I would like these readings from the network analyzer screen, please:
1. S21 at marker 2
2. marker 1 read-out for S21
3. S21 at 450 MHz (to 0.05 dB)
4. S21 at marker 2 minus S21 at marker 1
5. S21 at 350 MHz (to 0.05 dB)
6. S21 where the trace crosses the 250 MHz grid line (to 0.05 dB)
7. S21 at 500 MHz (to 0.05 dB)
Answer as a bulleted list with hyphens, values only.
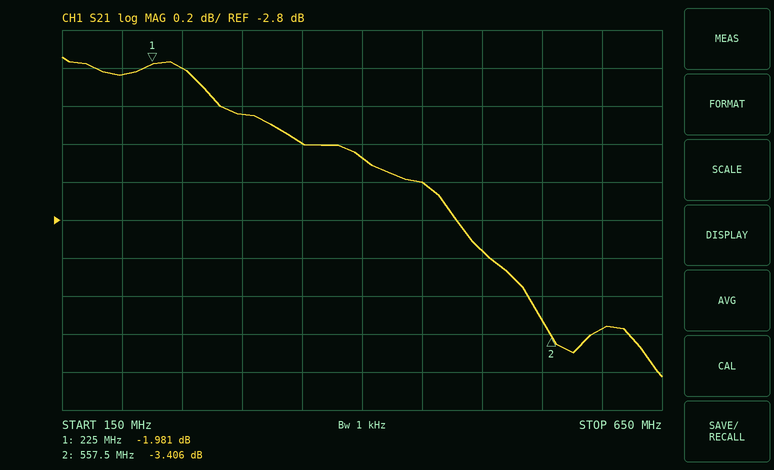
- -3.406 dB
- -1.981 dB
- -2.60 dB
- -1.425 dB
- -2.40 dB
- -2.00 dB
- -2.95 dB
